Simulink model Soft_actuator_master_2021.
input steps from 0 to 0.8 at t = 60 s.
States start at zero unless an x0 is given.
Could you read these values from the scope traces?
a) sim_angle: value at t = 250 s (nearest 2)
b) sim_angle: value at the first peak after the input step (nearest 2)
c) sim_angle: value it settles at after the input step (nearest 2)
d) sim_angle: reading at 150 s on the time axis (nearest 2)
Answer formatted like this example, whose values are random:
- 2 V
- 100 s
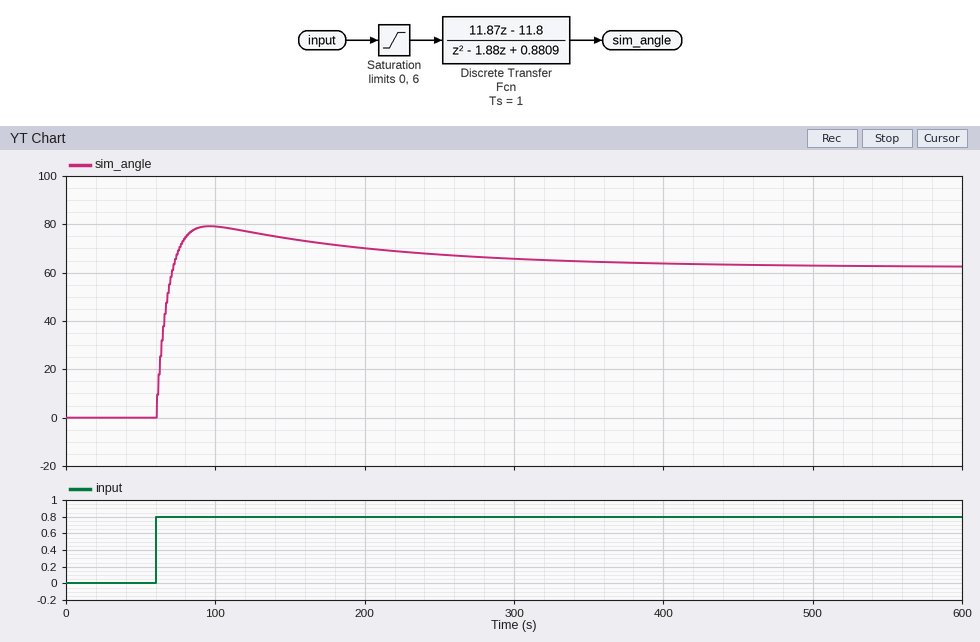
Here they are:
- 68
- 80
- 62
- 74
